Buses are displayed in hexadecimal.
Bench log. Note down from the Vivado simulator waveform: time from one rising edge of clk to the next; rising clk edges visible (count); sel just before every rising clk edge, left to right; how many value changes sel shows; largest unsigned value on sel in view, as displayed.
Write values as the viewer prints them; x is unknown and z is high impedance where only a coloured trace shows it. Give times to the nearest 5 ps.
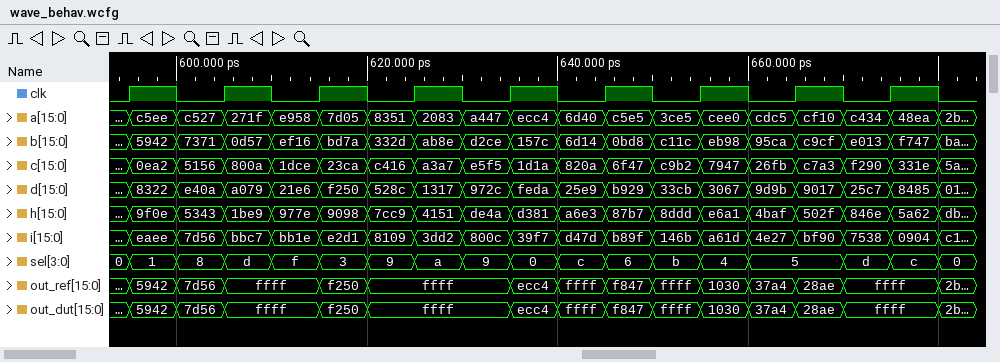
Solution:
10 ps
9
0, 8, f, 9, 9, c, b, 5, d
17
f
